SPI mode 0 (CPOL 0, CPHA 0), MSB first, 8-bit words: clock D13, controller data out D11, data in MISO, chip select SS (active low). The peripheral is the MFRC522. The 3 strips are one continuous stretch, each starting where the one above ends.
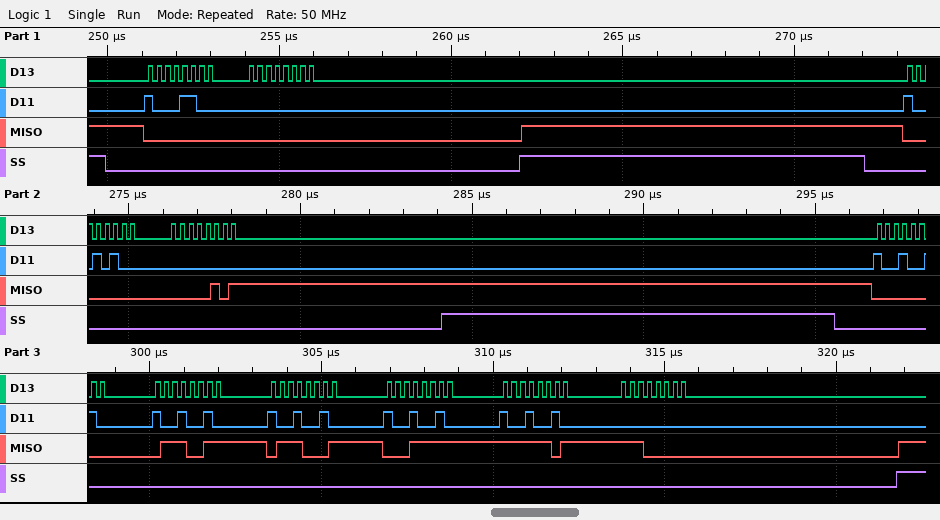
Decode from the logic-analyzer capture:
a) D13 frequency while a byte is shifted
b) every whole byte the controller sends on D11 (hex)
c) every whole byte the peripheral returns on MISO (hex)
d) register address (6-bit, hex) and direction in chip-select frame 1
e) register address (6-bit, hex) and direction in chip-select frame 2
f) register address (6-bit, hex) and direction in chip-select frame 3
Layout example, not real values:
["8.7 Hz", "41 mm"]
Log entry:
["4 MHz", "8C 00 94 00 92 92 92 92 92 00", "00 00 00 05 00 73 71 1F FD E0", "0x06 read", "0x0A read", "0x09 read"]
